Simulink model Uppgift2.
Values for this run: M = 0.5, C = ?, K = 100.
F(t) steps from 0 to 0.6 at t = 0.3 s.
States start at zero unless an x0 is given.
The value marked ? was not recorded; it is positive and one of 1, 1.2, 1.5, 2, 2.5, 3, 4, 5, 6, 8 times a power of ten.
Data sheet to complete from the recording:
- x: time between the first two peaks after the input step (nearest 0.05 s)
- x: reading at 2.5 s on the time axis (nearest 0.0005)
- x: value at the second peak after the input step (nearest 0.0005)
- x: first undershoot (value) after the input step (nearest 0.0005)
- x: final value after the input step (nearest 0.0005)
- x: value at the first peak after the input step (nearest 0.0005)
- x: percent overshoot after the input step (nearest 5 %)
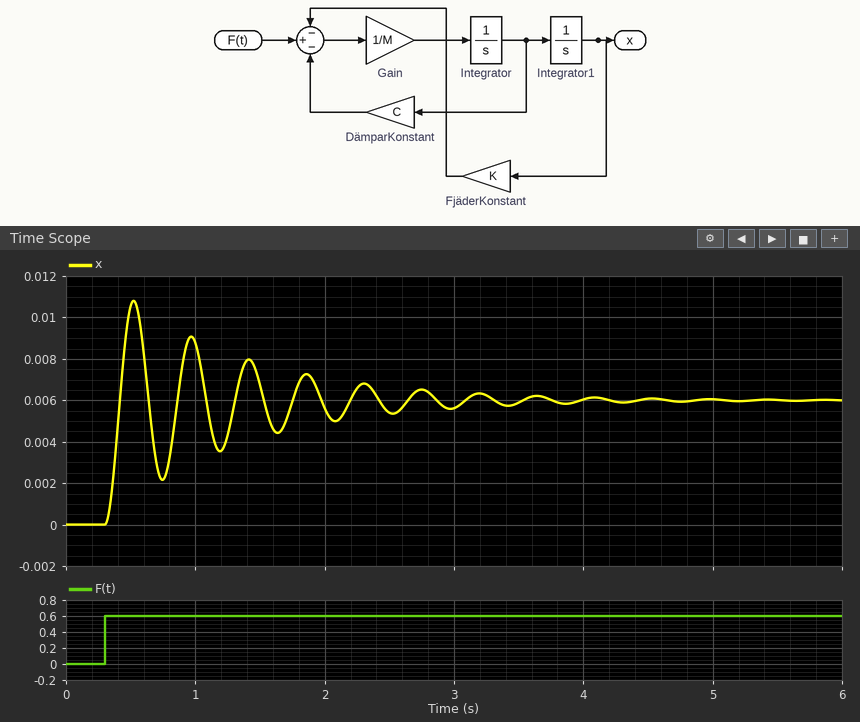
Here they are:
0.45 s
0.0055
0.0090
0.0020
0.0060
0.0110
80 %
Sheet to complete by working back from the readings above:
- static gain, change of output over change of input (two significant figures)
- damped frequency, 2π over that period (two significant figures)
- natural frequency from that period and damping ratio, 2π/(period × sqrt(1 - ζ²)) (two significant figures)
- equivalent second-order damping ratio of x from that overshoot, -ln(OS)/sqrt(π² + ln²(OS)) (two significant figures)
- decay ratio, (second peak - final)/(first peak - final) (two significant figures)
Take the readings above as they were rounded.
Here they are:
0.010
14 rad/s
14 rad/s
0.071
0.60
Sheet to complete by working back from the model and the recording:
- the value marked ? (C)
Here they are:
1
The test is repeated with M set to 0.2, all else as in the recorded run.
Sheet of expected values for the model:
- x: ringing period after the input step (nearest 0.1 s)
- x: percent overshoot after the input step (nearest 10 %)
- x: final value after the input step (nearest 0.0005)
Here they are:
0.3 s
70 %
0.0060
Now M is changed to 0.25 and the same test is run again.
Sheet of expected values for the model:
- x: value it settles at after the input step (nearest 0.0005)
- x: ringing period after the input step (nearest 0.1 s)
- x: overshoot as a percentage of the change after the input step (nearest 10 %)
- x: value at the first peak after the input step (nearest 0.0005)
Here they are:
0.0060
0.3 s
70 %
0.0105
